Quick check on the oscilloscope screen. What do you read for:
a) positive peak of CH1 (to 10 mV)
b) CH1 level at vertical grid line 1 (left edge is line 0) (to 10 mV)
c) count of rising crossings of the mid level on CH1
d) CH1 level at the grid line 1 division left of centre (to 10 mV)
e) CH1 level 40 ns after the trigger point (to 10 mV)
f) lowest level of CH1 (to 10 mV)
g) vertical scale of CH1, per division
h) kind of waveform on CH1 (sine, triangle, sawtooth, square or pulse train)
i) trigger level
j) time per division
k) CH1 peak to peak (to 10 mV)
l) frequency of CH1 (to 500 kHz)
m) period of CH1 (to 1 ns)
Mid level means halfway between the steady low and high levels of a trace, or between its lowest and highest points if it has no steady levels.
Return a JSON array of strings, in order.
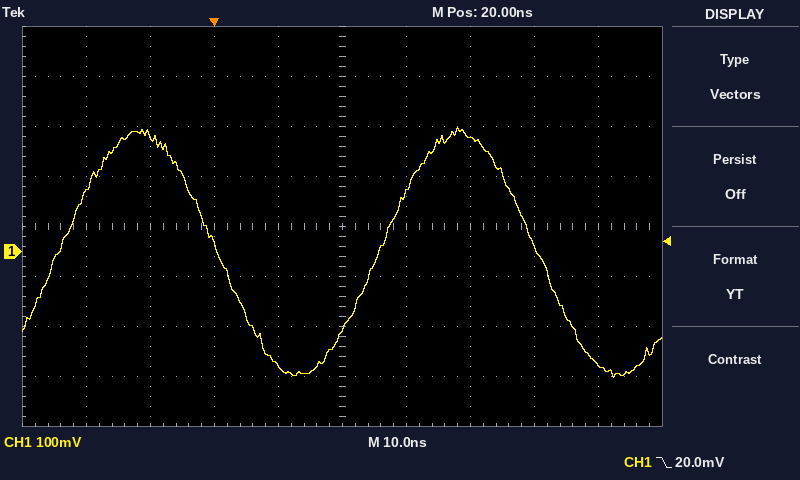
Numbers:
["250 mV", "120 mV", "2", "-230 mV", "230 mV", "-250 mV", "100 mV", "sine", "20.0 mV", "10 ns", "500 mV", "20.0 MHz", "50 ns"]
